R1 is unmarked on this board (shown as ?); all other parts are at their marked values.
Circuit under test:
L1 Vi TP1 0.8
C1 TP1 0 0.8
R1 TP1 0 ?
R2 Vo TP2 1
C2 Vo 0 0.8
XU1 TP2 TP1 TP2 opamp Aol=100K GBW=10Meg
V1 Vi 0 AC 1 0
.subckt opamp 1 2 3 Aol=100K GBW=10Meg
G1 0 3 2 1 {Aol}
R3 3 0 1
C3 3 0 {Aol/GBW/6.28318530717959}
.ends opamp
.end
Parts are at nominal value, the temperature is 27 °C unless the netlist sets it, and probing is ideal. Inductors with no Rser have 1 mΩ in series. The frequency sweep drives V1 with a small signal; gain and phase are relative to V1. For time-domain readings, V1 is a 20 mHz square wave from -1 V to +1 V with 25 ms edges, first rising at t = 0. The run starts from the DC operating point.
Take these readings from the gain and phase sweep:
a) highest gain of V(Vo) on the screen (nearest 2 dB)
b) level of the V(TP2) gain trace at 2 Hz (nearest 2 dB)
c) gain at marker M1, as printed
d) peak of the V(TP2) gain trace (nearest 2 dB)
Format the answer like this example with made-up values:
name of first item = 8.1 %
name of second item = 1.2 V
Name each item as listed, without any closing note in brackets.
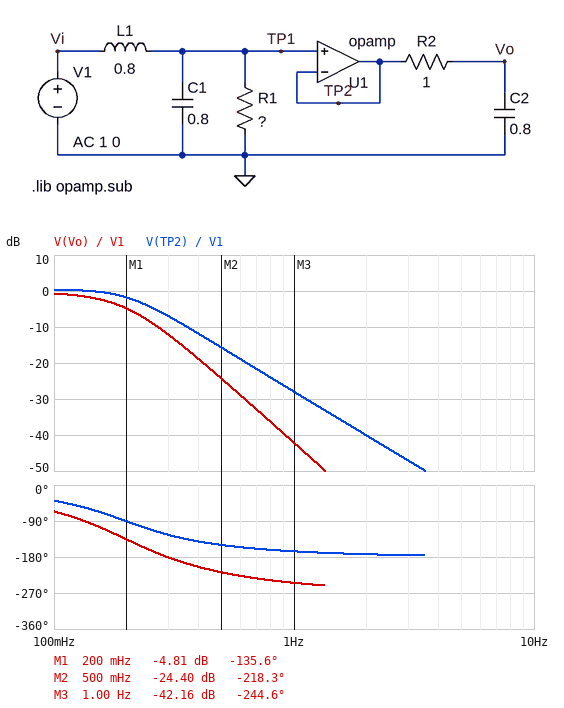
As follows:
highest gain of V(Vo) on the screen = 0 dB
level of the V(TP2) gain trace at 2 Hz = -40 dB
gain at marker M1, as printed = -4.81 dB
peak of the V(TP2) gain trace = 0 dB
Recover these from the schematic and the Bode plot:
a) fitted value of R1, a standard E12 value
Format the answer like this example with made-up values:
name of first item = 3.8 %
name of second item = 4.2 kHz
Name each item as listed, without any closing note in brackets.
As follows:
fitted value of R1, a standard E12 value = 0.82 Ω
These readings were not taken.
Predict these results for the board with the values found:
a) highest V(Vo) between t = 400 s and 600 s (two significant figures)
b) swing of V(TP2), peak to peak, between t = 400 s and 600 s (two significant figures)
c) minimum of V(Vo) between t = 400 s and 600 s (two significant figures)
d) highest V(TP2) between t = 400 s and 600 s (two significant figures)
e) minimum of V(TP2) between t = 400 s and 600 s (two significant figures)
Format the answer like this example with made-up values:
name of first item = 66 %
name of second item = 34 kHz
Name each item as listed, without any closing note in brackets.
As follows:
highest V(Vo) between t = 400 s and 600 s = 1.1 V
swing of V(TP2), peak to peak, between t = 400 s and 600 s = 2.4 V
minimum of V(Vo) between t = 400 s and 600 s = -1.1 V
highest V(TP2) between t = 400 s and 600 s = 1.2 V
minimum of V(TP2) between t = 400 s and 600 s = -1.2 V
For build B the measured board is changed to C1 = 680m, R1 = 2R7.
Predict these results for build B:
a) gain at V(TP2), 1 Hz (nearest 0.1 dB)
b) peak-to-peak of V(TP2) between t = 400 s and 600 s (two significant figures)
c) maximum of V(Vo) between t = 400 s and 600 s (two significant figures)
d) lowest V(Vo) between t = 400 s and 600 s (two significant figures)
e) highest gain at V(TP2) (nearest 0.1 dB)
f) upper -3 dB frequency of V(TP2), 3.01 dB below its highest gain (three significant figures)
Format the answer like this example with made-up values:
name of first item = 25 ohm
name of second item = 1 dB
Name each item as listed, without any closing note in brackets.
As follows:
gain at V(TP2), 1 Hz = -26.3 dB
peak-to-peak of V(TP2) between t = 400 s and 600 s = 4.1 V
maximum of V(Vo) between t = 400 s and 600 s = 1.6 V
lowest V(Vo) between t = 400 s and 600 s = -1.6 V
highest gain at V(TP2) = 8.1 dB
upper -3 dB frequency of V(TP2), 3.01 dB below its highest gain = 247 mHz
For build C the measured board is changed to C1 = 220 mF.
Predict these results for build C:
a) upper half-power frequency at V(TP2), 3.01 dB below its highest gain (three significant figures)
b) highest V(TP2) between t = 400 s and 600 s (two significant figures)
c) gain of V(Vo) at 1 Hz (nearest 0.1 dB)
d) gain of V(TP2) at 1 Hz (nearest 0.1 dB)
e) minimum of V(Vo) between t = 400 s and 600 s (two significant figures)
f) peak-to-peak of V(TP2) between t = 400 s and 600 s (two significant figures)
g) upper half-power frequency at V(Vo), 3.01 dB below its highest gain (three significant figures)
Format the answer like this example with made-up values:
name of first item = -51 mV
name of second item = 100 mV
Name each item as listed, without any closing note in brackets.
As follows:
upper half-power frequency at V(TP2), 3.01 dB below its highest gain = 198 mHz
highest V(TP2) between t = 400 s and 600 s = 1.0 V
gain of V(Vo) at 1 Hz = -32.8 dB
gain of V(TP2) at 1 Hz = -18.6 dB
minimum of V(Vo) between t = 400 s and 600 s = -1.0 V
peak-to-peak of V(TP2) between t = 400 s and 600 s = 2.0 V
upper half-power frequency at V(Vo), 3.01 dB below its highest gain = 129 mHz
